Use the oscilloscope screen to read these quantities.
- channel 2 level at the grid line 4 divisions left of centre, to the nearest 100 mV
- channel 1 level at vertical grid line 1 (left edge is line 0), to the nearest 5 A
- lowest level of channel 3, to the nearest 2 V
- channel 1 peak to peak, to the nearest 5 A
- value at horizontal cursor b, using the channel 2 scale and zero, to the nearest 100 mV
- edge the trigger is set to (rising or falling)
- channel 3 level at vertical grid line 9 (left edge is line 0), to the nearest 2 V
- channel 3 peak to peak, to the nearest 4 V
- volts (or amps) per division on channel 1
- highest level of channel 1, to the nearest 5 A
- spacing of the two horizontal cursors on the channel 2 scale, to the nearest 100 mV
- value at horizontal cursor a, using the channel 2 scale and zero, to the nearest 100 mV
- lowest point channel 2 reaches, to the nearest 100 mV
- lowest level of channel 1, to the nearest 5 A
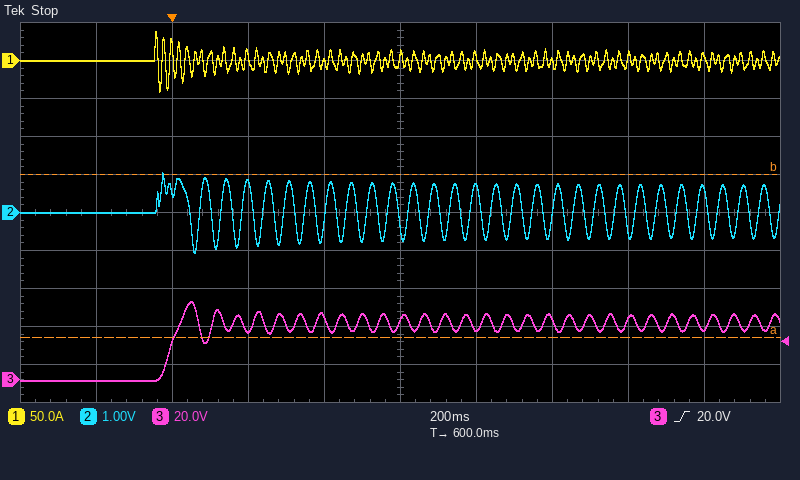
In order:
0.0 V
0 A
0 V
80 A
1.0 V
rising
28 V
40 V
50 A
40 A
4.3 V
-3.3 V
-1.1 V
-40 A
